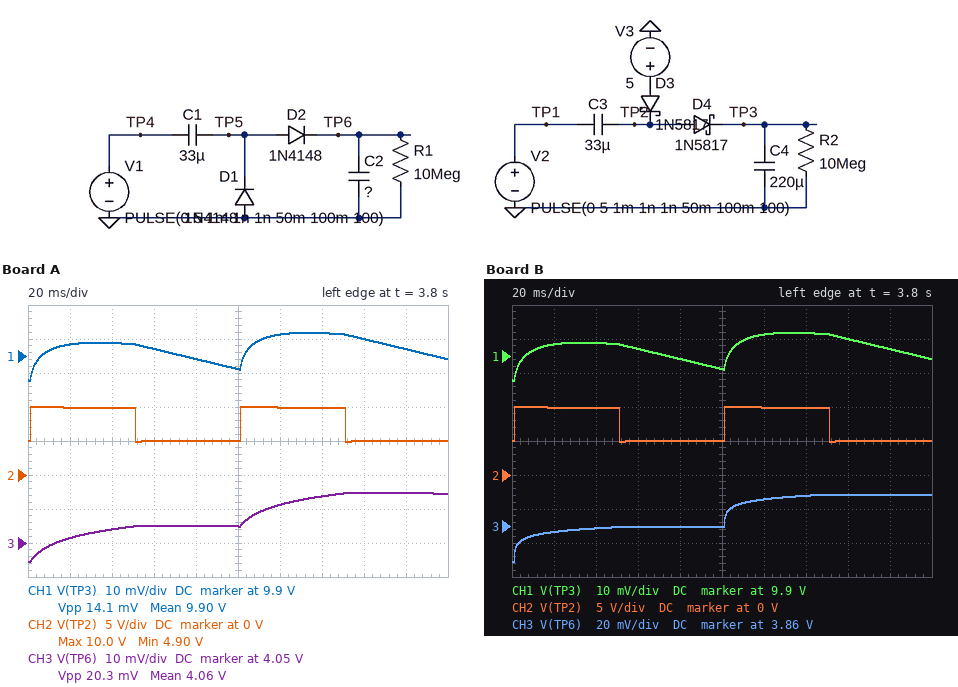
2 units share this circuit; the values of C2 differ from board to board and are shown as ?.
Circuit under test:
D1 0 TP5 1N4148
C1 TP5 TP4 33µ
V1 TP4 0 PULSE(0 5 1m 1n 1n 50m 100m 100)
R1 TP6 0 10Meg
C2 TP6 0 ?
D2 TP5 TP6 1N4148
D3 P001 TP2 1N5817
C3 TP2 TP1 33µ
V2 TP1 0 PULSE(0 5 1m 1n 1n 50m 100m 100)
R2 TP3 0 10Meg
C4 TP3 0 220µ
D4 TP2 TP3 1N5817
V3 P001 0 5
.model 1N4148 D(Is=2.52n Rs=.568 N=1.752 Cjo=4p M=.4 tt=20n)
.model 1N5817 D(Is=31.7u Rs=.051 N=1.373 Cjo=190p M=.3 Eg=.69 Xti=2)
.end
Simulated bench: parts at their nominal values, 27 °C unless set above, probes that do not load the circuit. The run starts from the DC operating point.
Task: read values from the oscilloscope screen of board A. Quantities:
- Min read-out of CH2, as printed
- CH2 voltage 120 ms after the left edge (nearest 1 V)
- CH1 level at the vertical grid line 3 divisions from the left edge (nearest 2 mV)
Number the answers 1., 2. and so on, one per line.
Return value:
1. 4.90 V
2. 10 V
3. 9.902 V
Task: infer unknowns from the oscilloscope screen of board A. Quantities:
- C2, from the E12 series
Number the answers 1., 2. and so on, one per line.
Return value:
1. 330 µF
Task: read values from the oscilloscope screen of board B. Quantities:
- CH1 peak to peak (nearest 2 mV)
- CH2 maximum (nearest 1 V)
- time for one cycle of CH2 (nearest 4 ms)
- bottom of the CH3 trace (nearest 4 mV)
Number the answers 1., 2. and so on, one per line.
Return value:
1. 14 mV
2. 10 V
3. 100 ms
4. 3.840 V
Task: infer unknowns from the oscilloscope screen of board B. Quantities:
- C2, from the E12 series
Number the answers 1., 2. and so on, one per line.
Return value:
1. 470 µF
